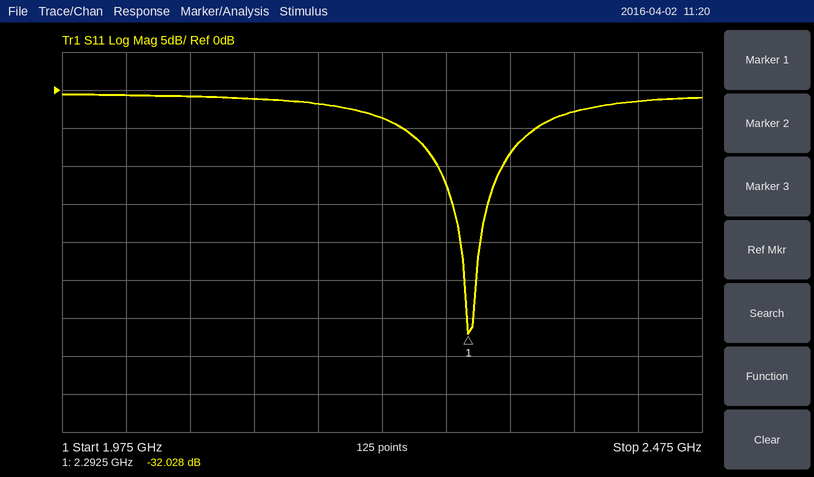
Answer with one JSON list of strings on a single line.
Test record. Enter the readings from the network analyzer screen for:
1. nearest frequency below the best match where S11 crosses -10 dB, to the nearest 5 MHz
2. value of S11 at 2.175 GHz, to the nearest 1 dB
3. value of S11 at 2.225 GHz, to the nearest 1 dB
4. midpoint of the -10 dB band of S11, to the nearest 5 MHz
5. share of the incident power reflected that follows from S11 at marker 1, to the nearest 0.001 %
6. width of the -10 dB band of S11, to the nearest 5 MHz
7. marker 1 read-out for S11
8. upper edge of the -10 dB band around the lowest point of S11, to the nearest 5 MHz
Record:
["2.270 GHz", "-2 dB", "-4 dB", "2.295 GHz", "0.063 %", "50 MHz", "-32.028 dB", "2.320 GHz"]
